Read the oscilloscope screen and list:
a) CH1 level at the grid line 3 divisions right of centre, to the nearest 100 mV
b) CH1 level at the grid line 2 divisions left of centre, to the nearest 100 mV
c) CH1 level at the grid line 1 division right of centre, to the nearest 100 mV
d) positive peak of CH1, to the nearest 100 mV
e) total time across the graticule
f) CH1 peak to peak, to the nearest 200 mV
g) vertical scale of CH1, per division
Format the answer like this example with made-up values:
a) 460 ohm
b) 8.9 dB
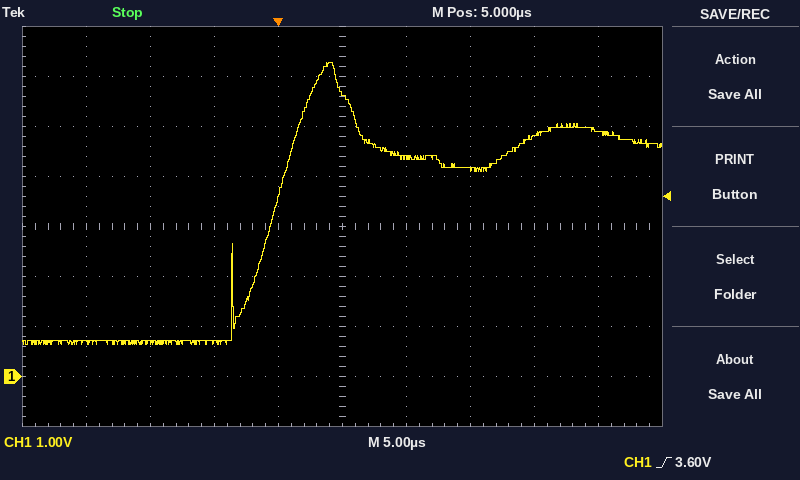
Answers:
a) 4.8 V
b) 700 mV
c) 4.4 V
d) 6.3 V
e) 50 µs
f) 5.6 V
g) 1 V
